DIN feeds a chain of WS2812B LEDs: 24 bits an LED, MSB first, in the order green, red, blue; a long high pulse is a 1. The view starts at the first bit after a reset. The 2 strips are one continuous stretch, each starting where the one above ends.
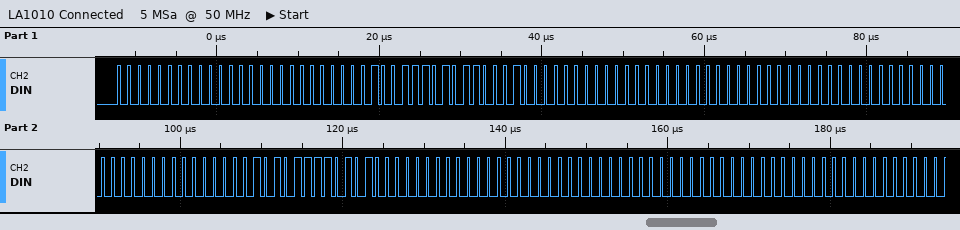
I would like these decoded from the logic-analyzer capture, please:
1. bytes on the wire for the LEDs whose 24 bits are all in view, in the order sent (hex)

00 00 00 4E B1 00 00 00 00 00 00 00 57 A8 00 00 00 00
